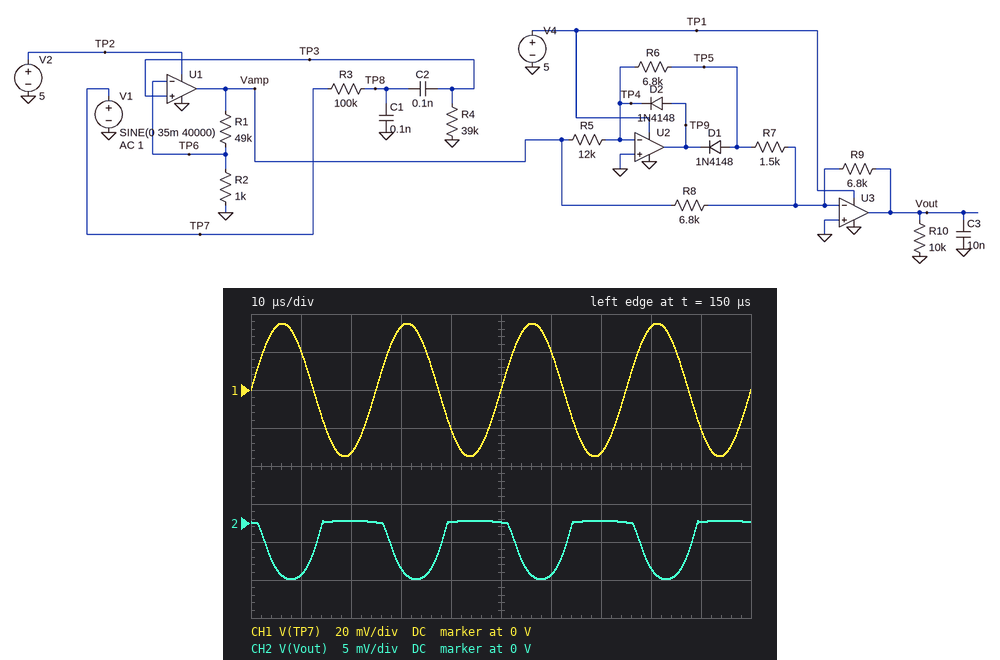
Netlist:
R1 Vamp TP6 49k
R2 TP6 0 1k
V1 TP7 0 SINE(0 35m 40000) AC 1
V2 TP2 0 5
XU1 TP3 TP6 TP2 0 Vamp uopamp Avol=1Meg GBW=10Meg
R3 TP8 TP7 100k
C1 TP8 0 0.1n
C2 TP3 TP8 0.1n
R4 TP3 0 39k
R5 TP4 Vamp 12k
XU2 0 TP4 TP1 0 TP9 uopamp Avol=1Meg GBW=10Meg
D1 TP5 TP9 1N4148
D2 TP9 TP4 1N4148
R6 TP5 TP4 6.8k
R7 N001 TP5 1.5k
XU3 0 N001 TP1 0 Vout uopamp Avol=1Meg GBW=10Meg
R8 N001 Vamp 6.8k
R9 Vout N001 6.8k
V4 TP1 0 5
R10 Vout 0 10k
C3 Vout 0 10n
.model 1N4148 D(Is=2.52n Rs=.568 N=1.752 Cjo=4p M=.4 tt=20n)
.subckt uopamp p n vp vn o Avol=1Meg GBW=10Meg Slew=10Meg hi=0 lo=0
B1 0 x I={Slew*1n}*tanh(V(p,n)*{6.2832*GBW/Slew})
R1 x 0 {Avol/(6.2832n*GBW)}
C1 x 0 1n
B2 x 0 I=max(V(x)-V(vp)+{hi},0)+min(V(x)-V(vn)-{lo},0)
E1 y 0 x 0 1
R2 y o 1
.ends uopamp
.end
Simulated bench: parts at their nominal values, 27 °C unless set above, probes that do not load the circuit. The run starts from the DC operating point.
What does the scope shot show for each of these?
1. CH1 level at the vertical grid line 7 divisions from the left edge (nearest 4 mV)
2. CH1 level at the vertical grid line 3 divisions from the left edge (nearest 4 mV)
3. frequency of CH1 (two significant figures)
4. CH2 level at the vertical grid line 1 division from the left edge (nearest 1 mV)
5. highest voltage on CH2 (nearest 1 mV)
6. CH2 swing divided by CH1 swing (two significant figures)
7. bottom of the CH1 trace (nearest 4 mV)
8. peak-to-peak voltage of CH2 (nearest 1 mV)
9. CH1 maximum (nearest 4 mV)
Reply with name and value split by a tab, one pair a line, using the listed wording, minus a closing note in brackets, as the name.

CH1 level at the vertical grid line 7 divisions from the left edge	-32 mV
CH1 level at the vertical grid line 3 divisions from the left edge	32 mV
frequency of CH1	40 kHz
CH2 level at the vertical grid line 1 division from the left edge	-7 mV
highest voltage on CH2	0 V
CH2 swing divided by CH1 swing	0.11
bottom of the CH1 trace	-36 mV
peak-to-peak voltage of CH2	8 mV
CH1 maximum	36 mV
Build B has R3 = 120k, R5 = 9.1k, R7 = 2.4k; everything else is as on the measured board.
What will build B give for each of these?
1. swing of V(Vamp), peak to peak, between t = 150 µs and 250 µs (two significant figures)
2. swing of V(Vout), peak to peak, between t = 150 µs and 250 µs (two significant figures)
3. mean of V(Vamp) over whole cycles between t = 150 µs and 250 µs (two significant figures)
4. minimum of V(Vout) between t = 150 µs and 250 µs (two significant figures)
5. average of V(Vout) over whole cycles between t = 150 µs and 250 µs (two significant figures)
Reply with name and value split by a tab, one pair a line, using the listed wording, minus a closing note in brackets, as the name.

swing of V(Vamp), peak to peak, between t = 150 µs and 250 µs	230 mV
swing of V(Vout), peak to peak, between t = 150 µs and 250 µs	7.0 mV
mean of V(Vamp) over whole cycles between t = 150 µs and 250 µs	74 mV
minimum of V(Vout) between t = 150 µs and 250 µs	-6.7 mV
average of V(Vout) over whole cycles between t = 150 µs and 250 µs	-2.2 mV
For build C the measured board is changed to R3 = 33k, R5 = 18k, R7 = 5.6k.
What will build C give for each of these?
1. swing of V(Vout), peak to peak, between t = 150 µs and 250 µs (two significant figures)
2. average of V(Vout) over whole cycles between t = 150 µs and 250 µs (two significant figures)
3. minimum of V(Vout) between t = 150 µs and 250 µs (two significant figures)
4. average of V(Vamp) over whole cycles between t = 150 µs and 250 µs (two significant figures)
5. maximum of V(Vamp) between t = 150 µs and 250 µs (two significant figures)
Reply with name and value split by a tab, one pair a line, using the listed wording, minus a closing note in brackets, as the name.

swing of V(Vout), peak to peak, between t = 150 µs and 250 µs	10 mV
average of V(Vout) over whole cycles between t = 150 µs and 250 µs	-3.7 mV
minimum of V(Vout) between t = 150 µs and 250 µs	-9.6 mV
average of V(Vamp) over whole cycles between t = 150 µs and 250 µs	200 mV
maximum of V(Vamp) between t = 150 µs and 250 µs	640 mV
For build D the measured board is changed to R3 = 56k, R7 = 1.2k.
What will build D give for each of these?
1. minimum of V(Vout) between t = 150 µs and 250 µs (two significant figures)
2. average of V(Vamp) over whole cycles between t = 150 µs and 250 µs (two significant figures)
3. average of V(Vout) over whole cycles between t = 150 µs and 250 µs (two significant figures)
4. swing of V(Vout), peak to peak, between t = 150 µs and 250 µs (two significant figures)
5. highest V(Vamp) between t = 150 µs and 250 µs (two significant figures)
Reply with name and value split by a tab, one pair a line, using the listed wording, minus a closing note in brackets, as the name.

minimum of V(Vout) between t = 150 µs and 250 µs	-9.1 mV
average of V(Vamp) over whole cycles between t = 150 µs and 250 µs	140 mV
average of V(Vout) over whole cycles between t = 150 µs and 250 µs	-3.3 mV
swing of V(Vout), peak to peak, between t = 150 µs and 250 µs	9.6 mV
highest V(Vamp) between t = 150 µs and 250 µs	440 mV
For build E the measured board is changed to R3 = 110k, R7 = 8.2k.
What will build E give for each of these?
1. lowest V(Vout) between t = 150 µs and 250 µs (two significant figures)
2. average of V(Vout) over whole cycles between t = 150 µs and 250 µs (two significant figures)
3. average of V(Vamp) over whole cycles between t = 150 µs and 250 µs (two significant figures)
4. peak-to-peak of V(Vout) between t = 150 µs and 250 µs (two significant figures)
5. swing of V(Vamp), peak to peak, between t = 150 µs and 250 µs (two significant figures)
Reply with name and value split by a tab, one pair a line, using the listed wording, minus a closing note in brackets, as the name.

lowest V(Vout) between t = 150 µs and 250 µs	-6.9 mV
average of V(Vout) over whole cycles between t = 150 µs and 250 µs	-2.3 mV
average of V(Vamp) over whole cycles between t = 150 µs and 250 µs	80 mV
peak-to-peak of V(Vout) between t = 150 µs and 250 µs	7.2 mV
swing of V(Vamp), peak to peak, between t = 150 µs and 250 µs	250 mV
